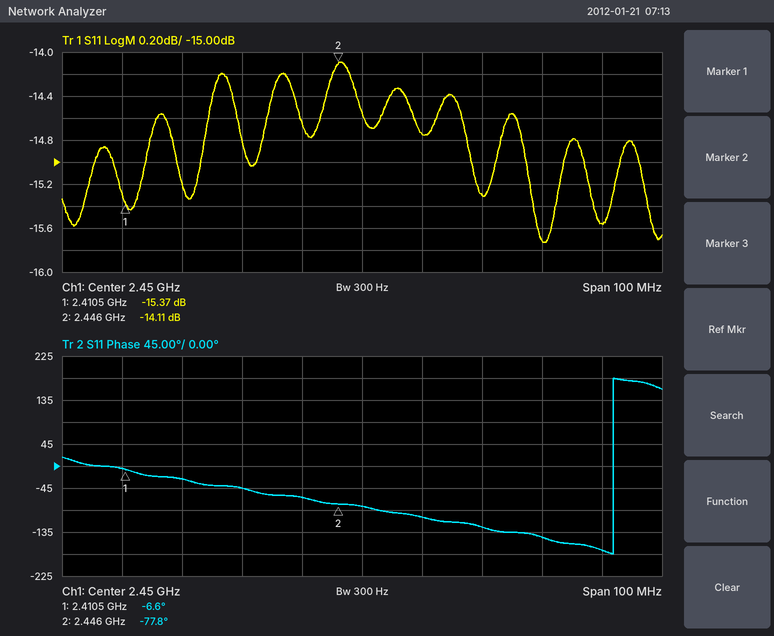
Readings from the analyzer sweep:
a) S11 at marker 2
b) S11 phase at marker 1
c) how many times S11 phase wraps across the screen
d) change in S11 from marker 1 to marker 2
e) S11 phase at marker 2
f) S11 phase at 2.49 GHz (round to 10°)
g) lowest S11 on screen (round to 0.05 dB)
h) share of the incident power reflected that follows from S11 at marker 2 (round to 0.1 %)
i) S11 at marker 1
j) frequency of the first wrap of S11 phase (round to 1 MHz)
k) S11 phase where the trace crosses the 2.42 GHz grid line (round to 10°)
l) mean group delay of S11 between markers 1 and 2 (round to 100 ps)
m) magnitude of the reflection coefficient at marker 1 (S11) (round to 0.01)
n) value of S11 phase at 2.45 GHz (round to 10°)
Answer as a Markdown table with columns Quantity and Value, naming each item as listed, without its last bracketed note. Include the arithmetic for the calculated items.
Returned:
| Quantity | Value |
|---|---|
| S11 at marker 2 | -14.11 dB |
| S11 phase at marker 1 | -6.6° |
| how many times S11 phase wraps across the screen | 1 |
| change in S11 from marker 1 to marker 2 | -14.11 − (-15.37) = 1.26 dB |
| S11 phase at marker 2 | -77.8° |
| S11 phase at 2.49 GHz | -170° |
| lowest S11 on screen | -15.75 dB |
| share of the incident power reflected that follows from S11 at marker 2 | 10^(-14.11/10) ≈ 3.9 % |
| S11 at marker 1 | -15.37 dB |
| frequency of the first wrap of S11 phase | 2.492 GHz |
| S11 phase where the trace crosses the 2.42 GHz grid line | -30° |
| mean group delay of S11 between markers 1 and 2 | −(-77.8° − (-6.6°))/(360° × 35.5 MHz) ≈ 5.6 ns |
| magnitude of the reflection coefficient at marker 1 (S11) | 10^(-15.37/20) ≈ 0.17 |
| value of S11 phase at 2.45 GHz | -80° |
